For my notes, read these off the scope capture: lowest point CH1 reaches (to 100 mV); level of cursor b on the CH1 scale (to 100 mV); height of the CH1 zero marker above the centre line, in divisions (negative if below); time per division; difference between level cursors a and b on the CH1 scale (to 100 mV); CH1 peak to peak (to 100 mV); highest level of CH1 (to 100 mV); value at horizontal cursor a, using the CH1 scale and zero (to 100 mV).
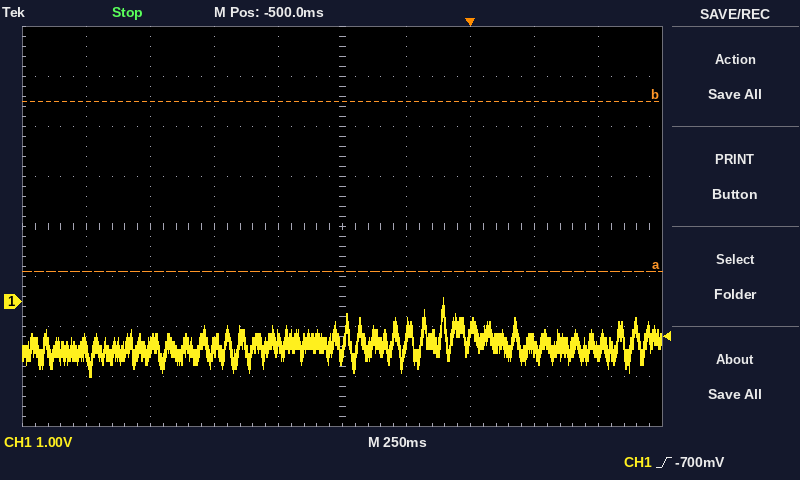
-1.5 V
4.0 V
-1.5 div
250 ms
3.4 V
1.6 V
100 mV
600 mV
